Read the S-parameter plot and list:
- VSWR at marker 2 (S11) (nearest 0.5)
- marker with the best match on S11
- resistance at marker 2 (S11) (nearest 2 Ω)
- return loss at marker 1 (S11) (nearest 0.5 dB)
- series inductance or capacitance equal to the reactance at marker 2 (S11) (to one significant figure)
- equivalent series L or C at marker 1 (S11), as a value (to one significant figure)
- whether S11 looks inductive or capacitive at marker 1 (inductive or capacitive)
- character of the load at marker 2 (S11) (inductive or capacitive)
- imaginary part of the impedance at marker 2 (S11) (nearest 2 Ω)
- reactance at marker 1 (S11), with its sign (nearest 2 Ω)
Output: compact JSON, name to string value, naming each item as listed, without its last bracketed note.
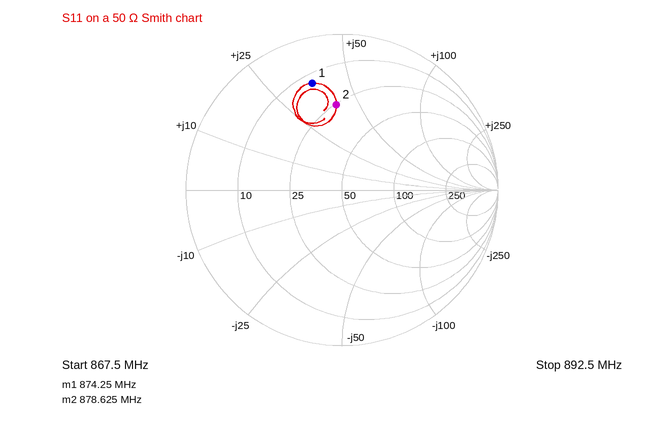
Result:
{"VSWR at marker 2 (S11)": "3.5", "marker with the best match on S11": "marker 2", "resistance at marker 2 (S11)": "26 Ω", "return loss at marker 1 (S11)": "3.0 dB", "series inductance or capacitance equal to the reactance at marker 2 (S11)": "7 nH", "equivalent series L or C at marker 1 (S11), as a value": "7 nH", "whether S11 looks inductive or capacitive at marker 1": "inductive", "character of the load at marker 2 (S11)": "inductive", "imaginary part of the impedance at marker 2 (S11)": "+40 Ω", "reactance at marker 1 (S11), with its sign": "+36 Ω"}
